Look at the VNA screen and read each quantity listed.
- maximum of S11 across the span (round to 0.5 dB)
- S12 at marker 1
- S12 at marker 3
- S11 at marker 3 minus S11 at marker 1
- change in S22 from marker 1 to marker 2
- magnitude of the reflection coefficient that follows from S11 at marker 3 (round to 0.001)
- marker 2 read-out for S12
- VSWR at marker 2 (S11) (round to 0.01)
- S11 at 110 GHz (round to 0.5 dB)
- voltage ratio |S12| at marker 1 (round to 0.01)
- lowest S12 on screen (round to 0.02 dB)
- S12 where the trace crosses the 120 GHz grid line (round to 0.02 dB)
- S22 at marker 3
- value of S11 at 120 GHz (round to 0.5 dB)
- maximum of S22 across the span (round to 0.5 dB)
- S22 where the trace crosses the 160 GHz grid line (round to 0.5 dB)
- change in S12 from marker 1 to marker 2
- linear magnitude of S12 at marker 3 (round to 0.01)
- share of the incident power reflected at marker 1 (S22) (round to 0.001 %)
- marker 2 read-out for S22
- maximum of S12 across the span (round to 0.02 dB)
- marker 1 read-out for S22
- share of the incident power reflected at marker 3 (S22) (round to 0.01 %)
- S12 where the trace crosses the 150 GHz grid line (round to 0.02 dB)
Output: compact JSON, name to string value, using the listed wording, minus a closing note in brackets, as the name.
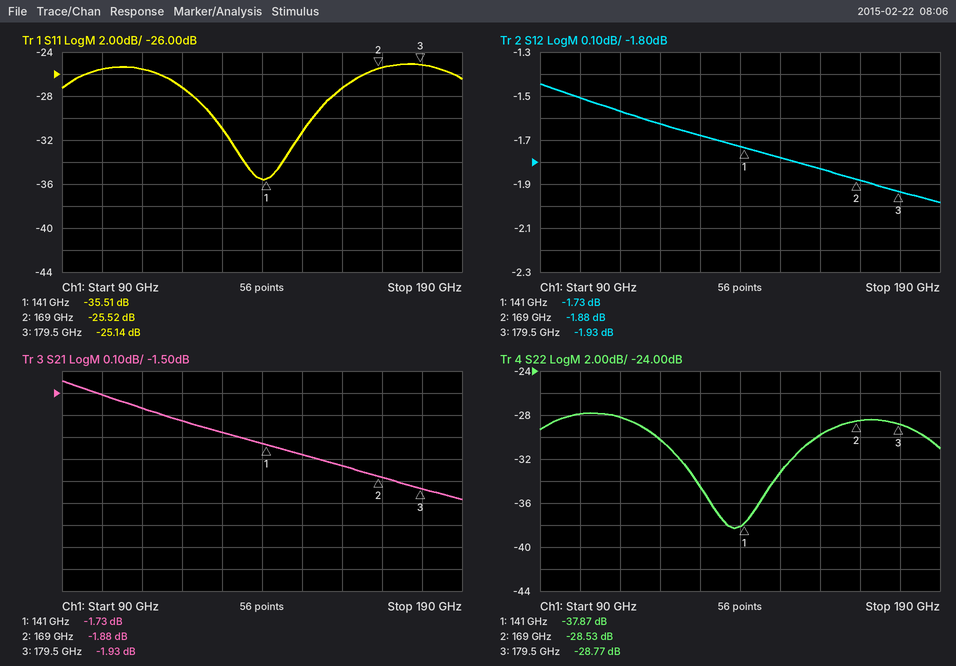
{"maximum of S11 across the span": "-25.0 dB", "S12 at marker 1": "-1.73 dB", "S12 at marker 3": "-1.93 dB", "S11 at marker 3 minus S11 at marker 1": "10.37 dB", "change in S22 from marker 1 to marker 2": "9.34 dB", "magnitude of the reflection coefficient that follows from S11 at marker 3": "0.055", "marker 2 read-out for S12": "-1.88 dB", "VSWR at marker 2 (S11)": "1.11", "S11 at 110 GHz": "-25.5 dB", "voltage ratio |S12| at marker 1": "0.82", "lowest S12 on screen": "-1.98 dB", "S12 where the trace crosses the 120 GHz grid line": "-1.62 dB", "S22 at marker 3": "-28.77 dB", "value of S11 at 120 GHz": "-27.0 dB", "maximum of S22 across the span": "-28.0 dB", "S22 where the trace crosses the 160 GHz grid line": "-30.0 dB", "change in S12 from marker 1 to marker 2": "-0.15 dB", "linear magnitude of S12 at marker 3": "0.80", "share of the incident power reflected at marker 1 (S22)": "0.016 %", "marker 2 read-out for S22": "-28.53 dB", "maximum of S12 across the span": "-1.44 dB", "marker 1 read-out for S22": "-37.87 dB", "share of the incident power reflected at marker 3 (S22)": "0.13 %", "S12 where the trace crosses the 150 GHz grid line": "-1.78 dB"}
